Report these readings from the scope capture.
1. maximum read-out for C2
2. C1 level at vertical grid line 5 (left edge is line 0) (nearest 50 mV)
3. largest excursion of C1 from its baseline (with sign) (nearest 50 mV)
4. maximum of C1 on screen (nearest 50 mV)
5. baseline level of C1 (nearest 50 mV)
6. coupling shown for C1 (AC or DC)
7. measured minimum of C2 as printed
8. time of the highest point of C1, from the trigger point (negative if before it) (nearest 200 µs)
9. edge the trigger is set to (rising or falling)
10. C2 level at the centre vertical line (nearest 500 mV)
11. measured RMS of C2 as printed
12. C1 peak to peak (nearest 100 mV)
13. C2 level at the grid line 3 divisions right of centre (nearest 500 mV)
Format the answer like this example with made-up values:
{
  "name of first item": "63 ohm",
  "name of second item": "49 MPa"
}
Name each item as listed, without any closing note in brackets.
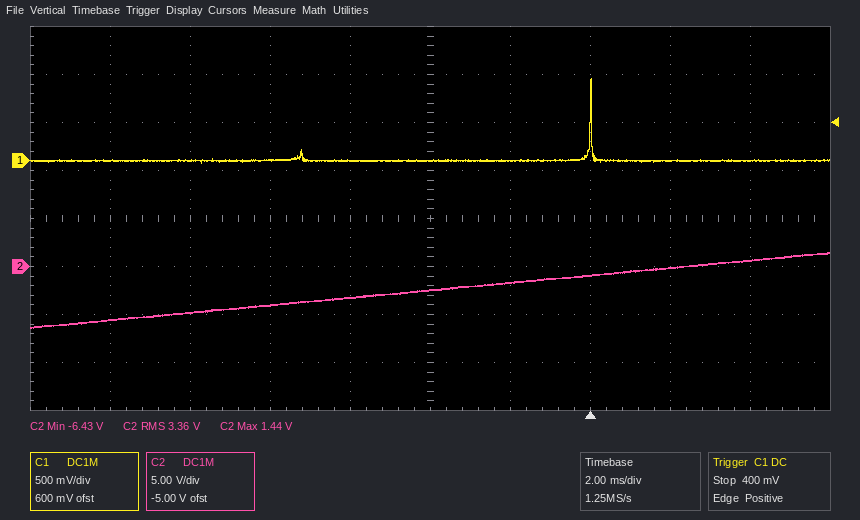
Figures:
{
  "maximum read-out for C2": "1.44 V",
  "C1 level at vertical grid line 5 (left edge is line 0)": "0 mV",
  "largest excursion of C1 from its baseline (with sign)": "+850 mV",
  "maximum of C1 on screen": "850 mV",
  "baseline level of C1": "0 mV",
  "coupling shown for C1": "DC",
  "measured minimum of C2 as printed": "-6.43 V",
  "time of the highest point of C1, from the trigger point (negative if before it)": "0.0 ms",
  "edge the trigger is set to": "rising",
  "C2 level at the centre vertical line": "-2.5 V",
  "measured RMS of C2 as printed": "3.36 V",
  "C1 peak to peak": "900 mV",
  "C2 level at the grid line 3 divisions right of centre": "0.0 V"
}
